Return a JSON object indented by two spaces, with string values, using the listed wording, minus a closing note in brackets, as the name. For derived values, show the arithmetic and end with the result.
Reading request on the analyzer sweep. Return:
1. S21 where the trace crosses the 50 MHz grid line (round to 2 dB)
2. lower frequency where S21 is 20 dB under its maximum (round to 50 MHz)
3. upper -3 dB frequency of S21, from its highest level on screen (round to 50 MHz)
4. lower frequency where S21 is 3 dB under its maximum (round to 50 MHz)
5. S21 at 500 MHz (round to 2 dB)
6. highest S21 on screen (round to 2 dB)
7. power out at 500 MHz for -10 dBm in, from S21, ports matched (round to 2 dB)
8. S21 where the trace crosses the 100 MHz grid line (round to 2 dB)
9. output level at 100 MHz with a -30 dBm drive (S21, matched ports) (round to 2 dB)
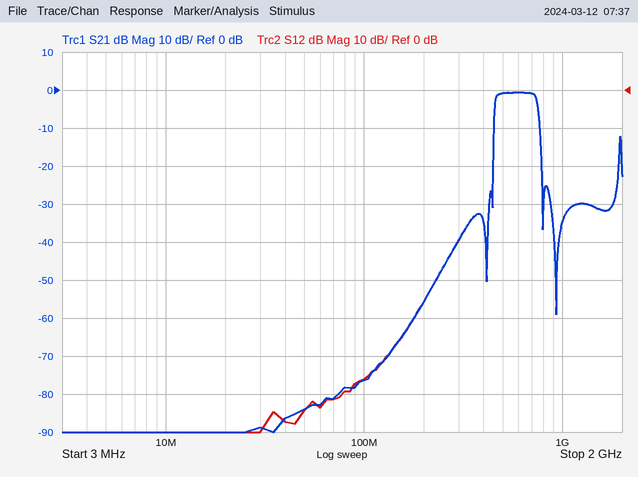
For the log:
{
  "S21 where the trace crosses the 50 MHz grid line": "-84 dB",
  "lower frequency where S21 is 20 dB under its maximum": "450 MHz",
  "upper -3 dB frequency of S21, from its highest level on screen": "750 MHz",
  "lower frequency where S21 is 3 dB under its maximum": "450 MHz",
  "S21 at 500 MHz": "0 dB",
  "highest S21 on screen": "0 dB",
  "power out at 500 MHz for -10 dBm in, from S21, ports matched": "-10 dBm + (0 dB) = -10 dBm",
  "S21 where the trace crosses the 100 MHz grid line": "-76 dB",
  "output level at 100 MHz with a -30 dBm drive (S21, matched ports)": "-30 dBm + (-76 dB) = -106 dBm"
}
